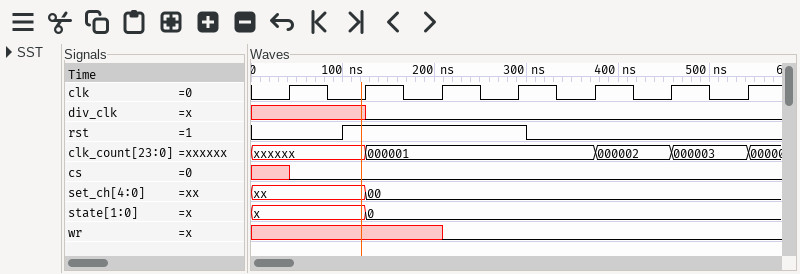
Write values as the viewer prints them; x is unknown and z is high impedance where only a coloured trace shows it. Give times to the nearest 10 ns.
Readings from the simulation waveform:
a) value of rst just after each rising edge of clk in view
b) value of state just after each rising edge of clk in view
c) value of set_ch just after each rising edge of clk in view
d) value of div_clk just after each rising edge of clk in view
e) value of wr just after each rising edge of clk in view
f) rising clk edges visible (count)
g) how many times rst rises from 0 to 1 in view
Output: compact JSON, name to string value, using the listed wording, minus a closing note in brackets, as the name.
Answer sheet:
{"value of rst just after each rising edge of clk in view": "0 1 1 1 0 0 0", "value of state just after each rising edge of clk in view": "x, 0, 0, 0, 0, 0, 0", "value of set_ch just after each rising edge of clk in view": "xx, 00, 00, 00, 00, 00, 00", "value of div_clk just after each rising edge of clk in view": "x 0 0 0 0 0 0", "value of wr just after each rising edge of clk in view": "x x 0 0 0 0 0", "rising clk edges visible": "7", "how many times rst rises from 0 to 1 in view": "1"}
